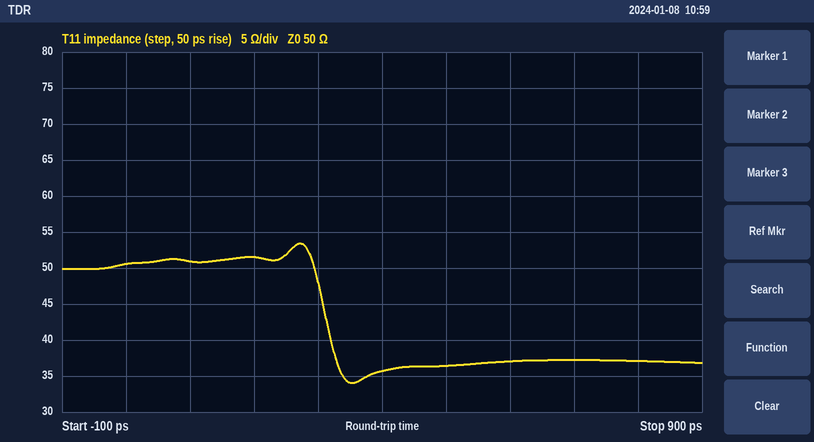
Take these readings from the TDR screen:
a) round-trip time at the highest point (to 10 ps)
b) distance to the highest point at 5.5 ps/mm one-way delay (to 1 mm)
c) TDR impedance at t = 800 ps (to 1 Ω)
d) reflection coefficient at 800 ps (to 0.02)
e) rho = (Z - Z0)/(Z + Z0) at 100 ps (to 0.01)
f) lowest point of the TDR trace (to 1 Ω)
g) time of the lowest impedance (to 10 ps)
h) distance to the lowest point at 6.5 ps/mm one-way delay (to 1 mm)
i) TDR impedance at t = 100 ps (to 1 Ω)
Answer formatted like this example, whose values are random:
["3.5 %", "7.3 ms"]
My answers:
["270 ps", "25 mm", "37 Ω", "-0.14", "+0.01", "34 Ω", "350 ps", "27 mm", "51 Ω"]
